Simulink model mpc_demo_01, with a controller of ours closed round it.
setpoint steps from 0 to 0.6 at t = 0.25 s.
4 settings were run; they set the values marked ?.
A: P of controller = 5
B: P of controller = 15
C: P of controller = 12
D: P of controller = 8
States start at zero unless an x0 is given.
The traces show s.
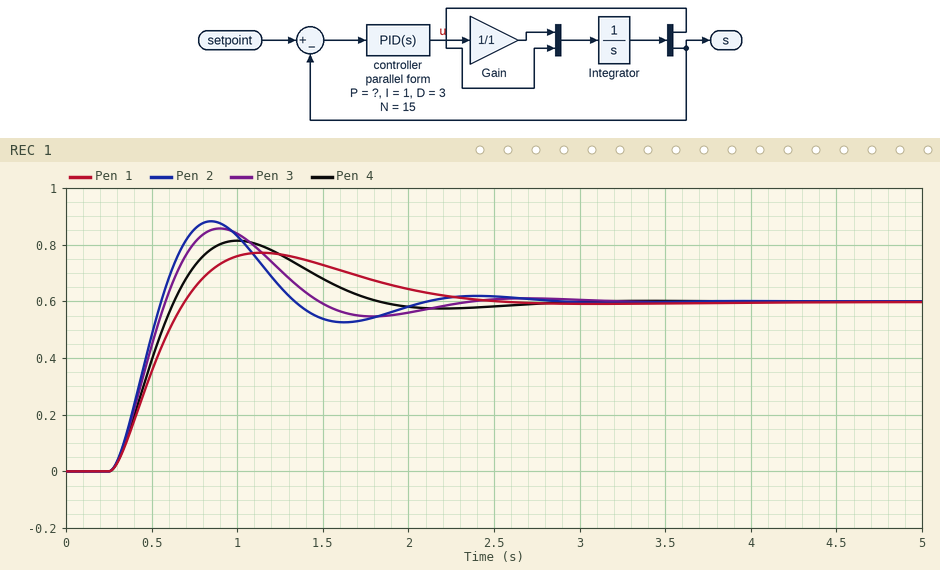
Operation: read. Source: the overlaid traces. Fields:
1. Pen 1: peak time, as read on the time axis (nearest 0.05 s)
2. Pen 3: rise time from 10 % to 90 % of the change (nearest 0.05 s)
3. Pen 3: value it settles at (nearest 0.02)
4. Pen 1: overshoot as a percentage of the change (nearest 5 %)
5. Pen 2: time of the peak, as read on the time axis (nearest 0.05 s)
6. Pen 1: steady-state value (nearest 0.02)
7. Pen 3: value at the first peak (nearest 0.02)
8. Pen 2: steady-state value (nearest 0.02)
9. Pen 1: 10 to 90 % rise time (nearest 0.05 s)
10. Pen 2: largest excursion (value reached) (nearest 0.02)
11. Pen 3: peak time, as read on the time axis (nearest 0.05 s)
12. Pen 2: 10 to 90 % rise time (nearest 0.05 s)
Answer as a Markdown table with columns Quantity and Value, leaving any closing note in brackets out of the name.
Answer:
| Quantity | Value |
|---|---|
| Pen 1: peak time, as read on the time axis | 1.15 s |
| Pen 3: rise time from 10 % to 90 % of the change | 0.25 s |
| Pen 3: value it settles at | 0.60 |
| Pen 1: overshoot as a percentage of the change | 30 % |
| Pen 2: time of the peak, as read on the time axis | 0.85 s |
| Pen 1: steady-state value | 0.60 |
| Pen 3: value at the first peak | 0.86 |
| Pen 2: steady-state value | 0.60 |
| Pen 1: 10 to 90 % rise time | 0.30 s |
| Pen 2: largest excursion (value reached) | 0.88 |
| Pen 3: peak time, as read on the time axis | 0.90 s |
| Pen 2: 10 to 90 % rise time | 0.20 s |
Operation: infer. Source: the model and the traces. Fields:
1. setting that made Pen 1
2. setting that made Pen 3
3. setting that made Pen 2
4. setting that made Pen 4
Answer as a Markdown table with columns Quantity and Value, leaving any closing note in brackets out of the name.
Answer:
| Quantity | Value |
|---|---|
| setting that made Pen 1 | A |
| setting that made Pen 3 | C |
| setting that made Pen 2 | B |
| setting that made Pen 4 | D |
